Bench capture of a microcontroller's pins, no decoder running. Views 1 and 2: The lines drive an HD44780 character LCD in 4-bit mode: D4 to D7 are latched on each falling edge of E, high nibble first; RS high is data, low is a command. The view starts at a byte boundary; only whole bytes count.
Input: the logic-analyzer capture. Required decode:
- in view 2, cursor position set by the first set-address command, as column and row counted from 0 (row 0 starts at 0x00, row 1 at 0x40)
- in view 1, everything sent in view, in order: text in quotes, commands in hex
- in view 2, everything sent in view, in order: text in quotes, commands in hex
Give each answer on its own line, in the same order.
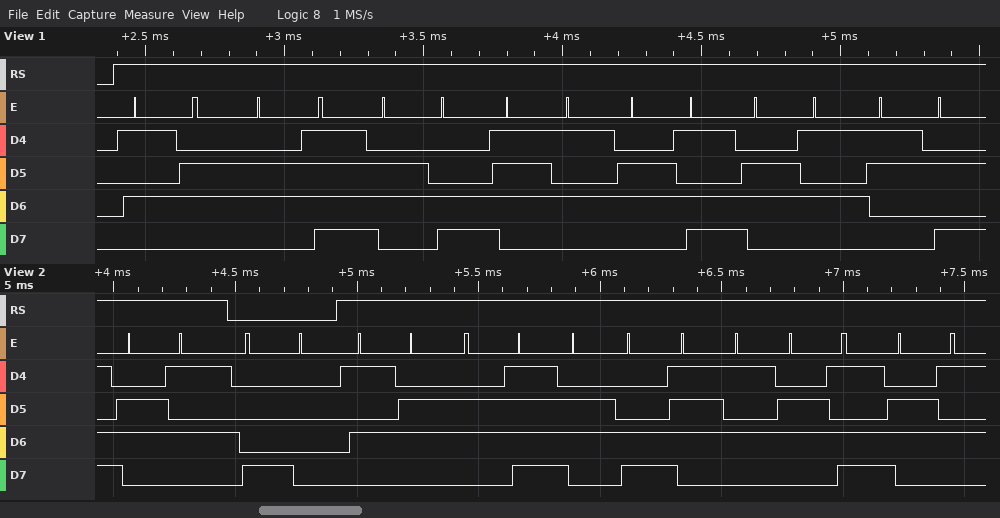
column 0, row 0
"Volume:"
"e" 0x80 "Volume"
